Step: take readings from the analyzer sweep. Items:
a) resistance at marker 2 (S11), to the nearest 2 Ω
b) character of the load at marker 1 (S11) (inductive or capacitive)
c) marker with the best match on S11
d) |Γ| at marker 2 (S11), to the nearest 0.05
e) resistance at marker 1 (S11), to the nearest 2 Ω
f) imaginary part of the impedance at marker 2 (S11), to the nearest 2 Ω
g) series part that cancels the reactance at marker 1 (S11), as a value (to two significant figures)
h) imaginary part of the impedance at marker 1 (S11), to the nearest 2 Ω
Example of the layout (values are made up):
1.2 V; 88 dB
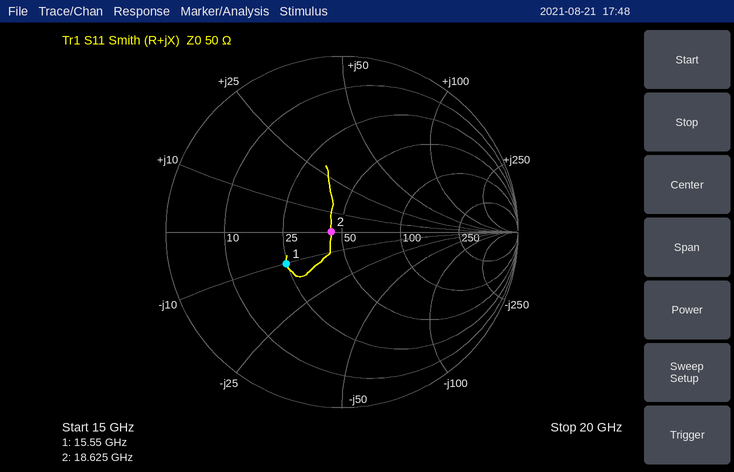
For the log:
44 Ω; capacitive; marker 2; 0.05; 24 Ω; 0 Ω; 100 pH; -10 Ω
